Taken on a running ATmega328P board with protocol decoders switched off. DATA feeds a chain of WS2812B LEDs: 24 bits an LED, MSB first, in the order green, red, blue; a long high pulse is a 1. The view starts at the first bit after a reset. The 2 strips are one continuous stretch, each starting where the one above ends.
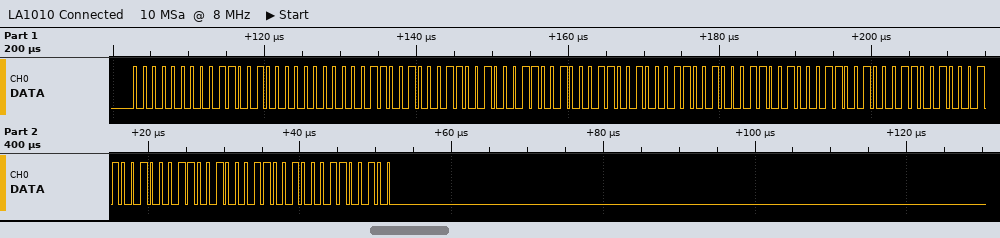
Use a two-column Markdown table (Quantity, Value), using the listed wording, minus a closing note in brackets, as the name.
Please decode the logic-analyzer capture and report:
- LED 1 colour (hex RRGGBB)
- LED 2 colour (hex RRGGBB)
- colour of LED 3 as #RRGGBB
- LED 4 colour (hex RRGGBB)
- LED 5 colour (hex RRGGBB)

| Quantity | Value |
|---|---|
| LED 1 colour | #640000 |
| LED 2 colour | #646464 |
| colour of LED 3 as #RRGGBB | #646464 |
| LED 4 colour | #646464 |
| LED 5 colour | #646464 |
